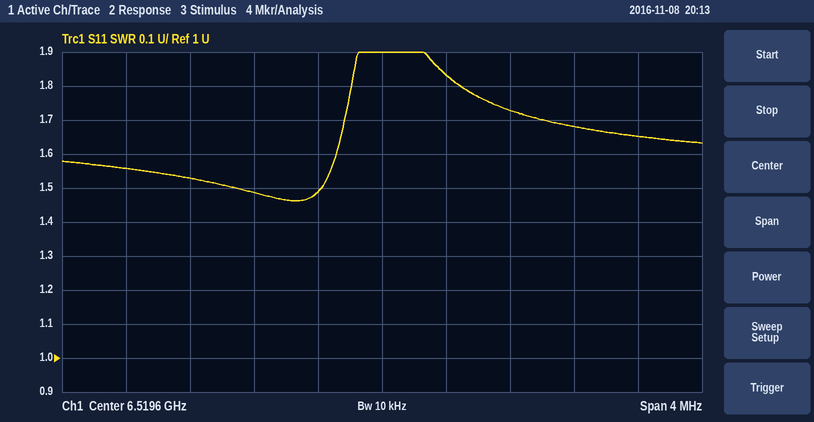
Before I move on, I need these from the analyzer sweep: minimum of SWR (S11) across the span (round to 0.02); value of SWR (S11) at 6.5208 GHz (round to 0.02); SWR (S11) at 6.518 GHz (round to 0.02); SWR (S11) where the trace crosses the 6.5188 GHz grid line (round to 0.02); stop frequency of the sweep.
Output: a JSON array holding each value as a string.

["1.46", "1.68", "1.56", "1.48", "6.5216 GHz"]
